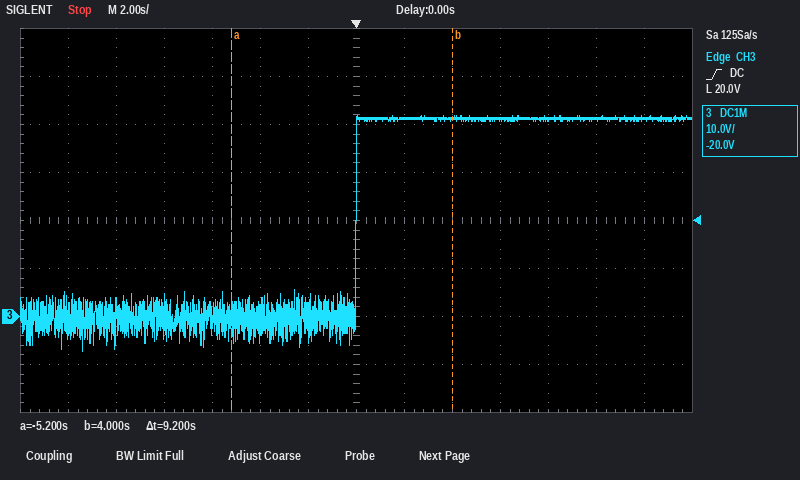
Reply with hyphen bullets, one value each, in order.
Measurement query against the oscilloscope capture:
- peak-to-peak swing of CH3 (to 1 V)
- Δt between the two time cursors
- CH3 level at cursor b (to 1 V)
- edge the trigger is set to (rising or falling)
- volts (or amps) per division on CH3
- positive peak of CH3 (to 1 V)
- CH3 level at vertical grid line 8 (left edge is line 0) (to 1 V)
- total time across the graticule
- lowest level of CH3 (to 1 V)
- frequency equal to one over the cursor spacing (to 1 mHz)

- 49 V
- 9.2 s
- 41 V
- rising
- 10 V
- 42 V
- 41 V
- 28 s
- -7 V
- 109 mHz
